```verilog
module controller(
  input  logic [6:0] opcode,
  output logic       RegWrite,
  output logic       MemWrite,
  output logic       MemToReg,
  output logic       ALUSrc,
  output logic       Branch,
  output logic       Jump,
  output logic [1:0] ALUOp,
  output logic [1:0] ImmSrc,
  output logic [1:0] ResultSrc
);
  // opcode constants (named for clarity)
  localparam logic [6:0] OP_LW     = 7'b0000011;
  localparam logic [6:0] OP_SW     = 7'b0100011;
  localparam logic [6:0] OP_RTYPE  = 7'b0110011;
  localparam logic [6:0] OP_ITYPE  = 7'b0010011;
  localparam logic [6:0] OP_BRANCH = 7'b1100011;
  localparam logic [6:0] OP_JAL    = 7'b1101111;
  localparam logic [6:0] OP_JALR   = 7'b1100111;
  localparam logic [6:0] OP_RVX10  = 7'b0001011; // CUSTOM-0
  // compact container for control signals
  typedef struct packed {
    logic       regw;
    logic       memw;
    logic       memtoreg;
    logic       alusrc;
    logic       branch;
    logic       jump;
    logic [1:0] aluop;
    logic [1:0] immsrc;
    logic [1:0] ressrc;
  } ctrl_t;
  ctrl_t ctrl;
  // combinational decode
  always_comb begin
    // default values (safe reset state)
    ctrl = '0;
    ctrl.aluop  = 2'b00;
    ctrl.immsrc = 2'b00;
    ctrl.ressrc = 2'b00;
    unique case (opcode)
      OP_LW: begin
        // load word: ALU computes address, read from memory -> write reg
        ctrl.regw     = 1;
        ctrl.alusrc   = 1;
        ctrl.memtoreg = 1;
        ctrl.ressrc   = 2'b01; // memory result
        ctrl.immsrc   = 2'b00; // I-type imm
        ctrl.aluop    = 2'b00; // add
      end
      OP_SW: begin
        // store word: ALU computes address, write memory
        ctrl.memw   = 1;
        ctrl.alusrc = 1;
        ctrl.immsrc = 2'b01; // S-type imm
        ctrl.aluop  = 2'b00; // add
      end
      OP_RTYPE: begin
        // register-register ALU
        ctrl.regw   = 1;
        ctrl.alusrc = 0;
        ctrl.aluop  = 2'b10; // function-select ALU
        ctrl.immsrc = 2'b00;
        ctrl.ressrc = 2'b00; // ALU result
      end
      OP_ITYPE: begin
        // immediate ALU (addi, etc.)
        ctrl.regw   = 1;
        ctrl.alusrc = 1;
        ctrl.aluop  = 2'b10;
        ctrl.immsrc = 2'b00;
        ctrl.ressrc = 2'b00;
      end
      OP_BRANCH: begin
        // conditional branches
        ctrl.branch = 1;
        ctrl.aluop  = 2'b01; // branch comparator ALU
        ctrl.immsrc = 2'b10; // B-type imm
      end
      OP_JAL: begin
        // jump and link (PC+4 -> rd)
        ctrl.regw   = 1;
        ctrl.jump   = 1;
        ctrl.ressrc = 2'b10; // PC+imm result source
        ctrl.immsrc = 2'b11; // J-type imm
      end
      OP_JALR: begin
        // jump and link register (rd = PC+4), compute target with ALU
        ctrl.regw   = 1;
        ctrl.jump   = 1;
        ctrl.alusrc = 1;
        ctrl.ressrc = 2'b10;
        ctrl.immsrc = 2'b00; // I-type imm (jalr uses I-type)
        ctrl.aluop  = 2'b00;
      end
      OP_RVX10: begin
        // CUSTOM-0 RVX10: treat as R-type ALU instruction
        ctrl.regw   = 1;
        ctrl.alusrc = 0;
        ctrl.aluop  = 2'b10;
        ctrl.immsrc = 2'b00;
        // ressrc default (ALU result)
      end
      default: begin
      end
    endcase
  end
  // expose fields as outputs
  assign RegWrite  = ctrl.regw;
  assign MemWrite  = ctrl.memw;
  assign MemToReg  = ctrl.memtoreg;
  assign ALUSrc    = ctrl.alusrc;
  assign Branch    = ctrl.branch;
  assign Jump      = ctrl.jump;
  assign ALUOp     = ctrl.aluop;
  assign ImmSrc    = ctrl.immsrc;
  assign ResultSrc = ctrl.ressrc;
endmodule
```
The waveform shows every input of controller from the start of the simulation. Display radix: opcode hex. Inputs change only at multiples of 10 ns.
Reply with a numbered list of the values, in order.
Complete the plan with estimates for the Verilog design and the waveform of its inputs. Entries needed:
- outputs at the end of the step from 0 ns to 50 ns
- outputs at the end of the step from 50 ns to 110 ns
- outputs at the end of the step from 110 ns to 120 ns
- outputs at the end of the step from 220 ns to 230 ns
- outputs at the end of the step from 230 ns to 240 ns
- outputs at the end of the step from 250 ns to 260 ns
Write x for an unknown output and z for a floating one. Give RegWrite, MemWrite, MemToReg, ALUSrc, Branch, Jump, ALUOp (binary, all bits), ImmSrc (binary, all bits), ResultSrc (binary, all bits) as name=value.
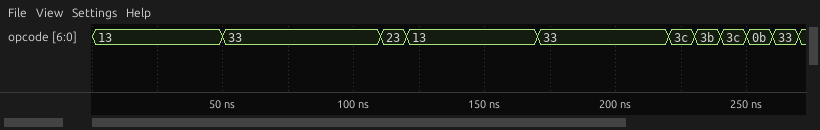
1. RegWrite=1, MemWrite=0, MemToReg=0, ALUSrc=1, Branch=0, Jump=0, ALUOp=10, ImmSrc=00, ResultSrc=00
2. RegWrite=1, MemWrite=0, MemToReg=0, ALUSrc=0, Branch=0, Jump=0, ALUOp=10, ImmSrc=00, ResultSrc=00
3. RegWrite=0, MemWrite=1, MemToReg=0, ALUSrc=1, Branch=0, Jump=0, ALUOp=00, ImmSrc=01, ResultSrc=00
4. RegWrite=0, MemWrite=0, MemToReg=0, ALUSrc=0, Branch=0, Jump=0, ALUOp=00, ImmSrc=00, ResultSrc=00
5. RegWrite=0, MemWrite=0, MemToReg=0, ALUSrc=0, Branch=0, Jump=0, ALUOp=00, ImmSrc=00, ResultSrc=00
6. RegWrite=1, MemWrite=0, MemToReg=0, ALUSrc=0, Branch=0, Jump=0, ALUOp=10, ImmSrc=00, ResultSrc=00
